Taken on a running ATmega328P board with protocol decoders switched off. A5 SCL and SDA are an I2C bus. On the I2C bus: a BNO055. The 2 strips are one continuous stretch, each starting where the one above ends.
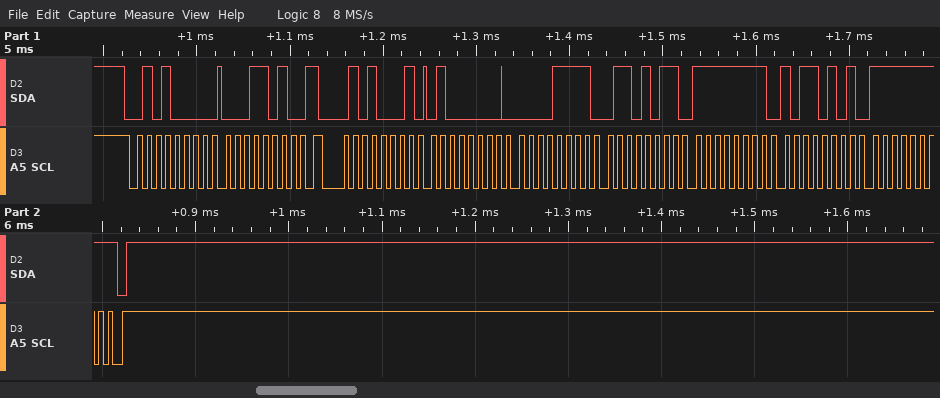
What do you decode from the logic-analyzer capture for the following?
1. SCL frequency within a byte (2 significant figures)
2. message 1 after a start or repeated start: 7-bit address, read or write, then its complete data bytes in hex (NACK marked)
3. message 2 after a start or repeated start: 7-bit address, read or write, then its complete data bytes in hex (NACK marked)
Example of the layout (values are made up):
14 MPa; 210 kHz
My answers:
100 kHz; 0x28 write: 1A; 0x28 read: 40 0F 6B FF B5 FF NACK
